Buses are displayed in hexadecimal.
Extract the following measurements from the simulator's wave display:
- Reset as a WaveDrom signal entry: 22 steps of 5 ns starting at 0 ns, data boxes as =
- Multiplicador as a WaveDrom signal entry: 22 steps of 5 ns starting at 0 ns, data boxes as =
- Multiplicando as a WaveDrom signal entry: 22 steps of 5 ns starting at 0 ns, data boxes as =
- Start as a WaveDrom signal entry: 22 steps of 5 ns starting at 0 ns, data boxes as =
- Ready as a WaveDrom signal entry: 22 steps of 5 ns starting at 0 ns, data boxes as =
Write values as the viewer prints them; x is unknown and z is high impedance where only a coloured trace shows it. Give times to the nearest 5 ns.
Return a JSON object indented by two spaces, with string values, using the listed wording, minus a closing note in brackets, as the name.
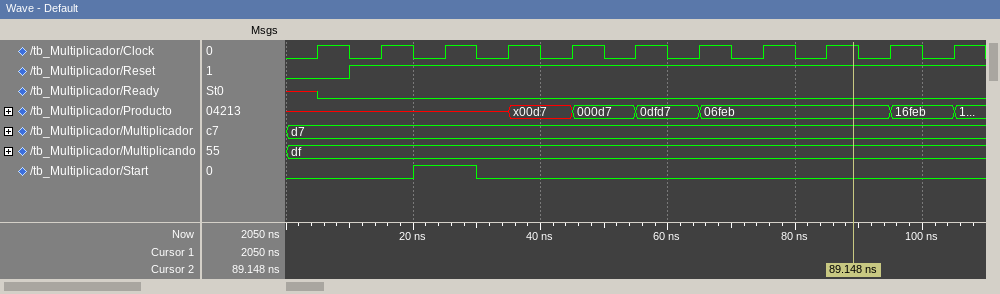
{
  "Reset as a WaveDrom signal entry: 22 steps of 5 ns starting at 0 ns, data boxes as =": "{name: 'Reset', wave: '0.1...................'}",
  "Multiplicador as a WaveDrom signal entry: 22 steps of 5 ns starting at 0 ns, data boxes as =": "{name: 'Multiplicador', wave: '=.....................', data: 'd7'}",
  "Multiplicando as a WaveDrom signal entry: 22 steps of 5 ns starting at 0 ns, data boxes as =": "{name: 'Multiplicando', wave: '=.....................', data: 'df'}",
  "Start as a WaveDrom signal entry: 22 steps of 5 ns starting at 0 ns, data boxes as =": "{name: 'Start', wave: '0...1.0...............'}",
  "Ready as a WaveDrom signal entry: 22 steps of 5 ns starting at 0 ns, data boxes as =": "{name: 'Ready', wave: 'x0....................'}"
}
